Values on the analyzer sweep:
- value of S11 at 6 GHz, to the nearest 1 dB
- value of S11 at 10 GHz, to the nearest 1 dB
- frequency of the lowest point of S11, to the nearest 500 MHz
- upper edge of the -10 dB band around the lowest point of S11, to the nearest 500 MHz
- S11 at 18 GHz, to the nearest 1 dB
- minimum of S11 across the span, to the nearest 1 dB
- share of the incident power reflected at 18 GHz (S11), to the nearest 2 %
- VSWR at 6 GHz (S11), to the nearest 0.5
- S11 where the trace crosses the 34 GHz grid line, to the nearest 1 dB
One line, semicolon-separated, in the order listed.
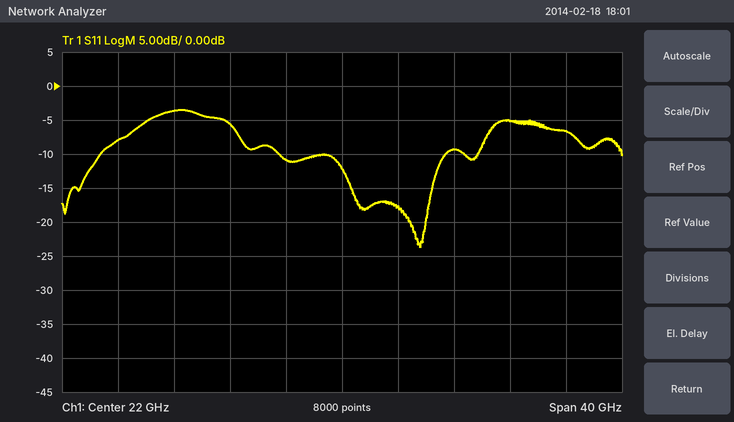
-8 dB; -4 dB; 27.5 GHz; 29.5 GHz; -11 dB; -24 dB; 8 %; 2.5; -5 dB
